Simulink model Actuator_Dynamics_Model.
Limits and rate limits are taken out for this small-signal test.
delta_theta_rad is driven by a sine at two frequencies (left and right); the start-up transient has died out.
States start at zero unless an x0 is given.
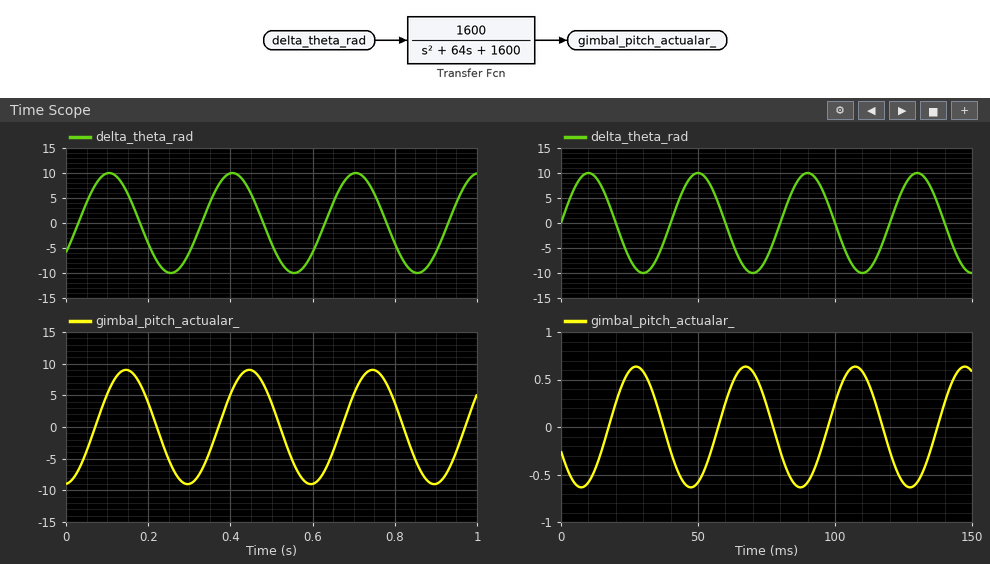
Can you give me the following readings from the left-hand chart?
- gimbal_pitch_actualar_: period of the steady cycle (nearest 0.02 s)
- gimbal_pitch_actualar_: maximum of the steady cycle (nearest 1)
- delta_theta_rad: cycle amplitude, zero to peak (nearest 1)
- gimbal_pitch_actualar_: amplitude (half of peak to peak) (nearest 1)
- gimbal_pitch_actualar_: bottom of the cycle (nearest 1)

0.30 s
9
10
9
-9
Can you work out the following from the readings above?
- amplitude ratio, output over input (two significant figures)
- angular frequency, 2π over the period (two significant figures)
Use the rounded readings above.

0.90
21 rad/s
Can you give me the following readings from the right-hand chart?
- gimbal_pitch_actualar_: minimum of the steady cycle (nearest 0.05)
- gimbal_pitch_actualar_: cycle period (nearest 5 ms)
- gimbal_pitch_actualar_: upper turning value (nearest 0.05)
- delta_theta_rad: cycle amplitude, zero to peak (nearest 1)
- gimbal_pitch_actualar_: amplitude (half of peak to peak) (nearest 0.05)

-0.65
40 ms
0.65
10
0.65
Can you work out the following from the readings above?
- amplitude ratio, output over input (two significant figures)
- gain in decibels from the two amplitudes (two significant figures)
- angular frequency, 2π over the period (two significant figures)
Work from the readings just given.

0.065
-24 dB
0.16 rad/ms
